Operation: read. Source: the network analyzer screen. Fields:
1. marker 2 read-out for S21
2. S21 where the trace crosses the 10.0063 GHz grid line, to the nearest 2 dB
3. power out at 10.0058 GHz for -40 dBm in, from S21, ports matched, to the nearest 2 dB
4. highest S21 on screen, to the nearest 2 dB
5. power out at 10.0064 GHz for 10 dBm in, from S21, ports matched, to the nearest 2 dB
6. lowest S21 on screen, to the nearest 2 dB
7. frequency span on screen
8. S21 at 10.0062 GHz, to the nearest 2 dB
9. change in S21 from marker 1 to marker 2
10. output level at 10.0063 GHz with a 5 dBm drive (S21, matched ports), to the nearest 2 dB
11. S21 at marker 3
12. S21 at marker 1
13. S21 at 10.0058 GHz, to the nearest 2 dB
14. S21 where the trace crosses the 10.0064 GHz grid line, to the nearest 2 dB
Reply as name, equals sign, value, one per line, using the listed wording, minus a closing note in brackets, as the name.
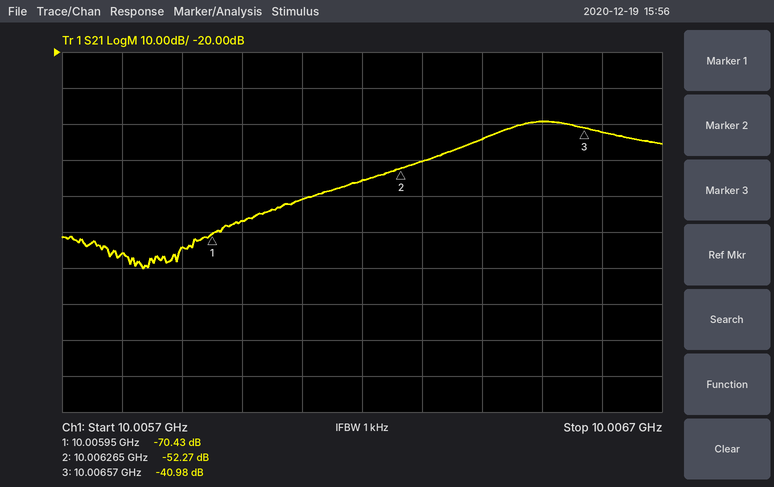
marker 2 read-out for S21 = -52.27 dB
S21 where the trace crosses the 10.0063 GHz grid line, to the nearest 2 dB = -50 dB
power out at 10.0058 GHz for -40 dBm in, from S21, ports matched, to the nearest 2 dB = -116 dBm
highest S21 on screen, to the nearest 2 dB = -40 dB
power out at 10.0064 GHz for 10 dBm in, from S21, ports matched, to the nearest 2 dB = -34 dBm
lowest S21 on screen, to the nearest 2 dB = -80 dB
frequency span on screen = 1 MHz
S21 at 10.0062 GHz, to the nearest 2 dB = -56 dB
change in S21 from marker 1 to marker 2 = 18.16 dB
output level at 10.0063 GHz with a 5 dBm drive (S21, matched ports), to the nearest 2 dB = -46 dBm
S21 at marker 3 = -40.98 dB
S21 at marker 1 = -70.43 dB
S21 at 10.0058 GHz, to the nearest 2 dB = -76 dB
S21 where the trace crosses the 10.0064 GHz grid line, to the nearest 2 dB = -44 dB
